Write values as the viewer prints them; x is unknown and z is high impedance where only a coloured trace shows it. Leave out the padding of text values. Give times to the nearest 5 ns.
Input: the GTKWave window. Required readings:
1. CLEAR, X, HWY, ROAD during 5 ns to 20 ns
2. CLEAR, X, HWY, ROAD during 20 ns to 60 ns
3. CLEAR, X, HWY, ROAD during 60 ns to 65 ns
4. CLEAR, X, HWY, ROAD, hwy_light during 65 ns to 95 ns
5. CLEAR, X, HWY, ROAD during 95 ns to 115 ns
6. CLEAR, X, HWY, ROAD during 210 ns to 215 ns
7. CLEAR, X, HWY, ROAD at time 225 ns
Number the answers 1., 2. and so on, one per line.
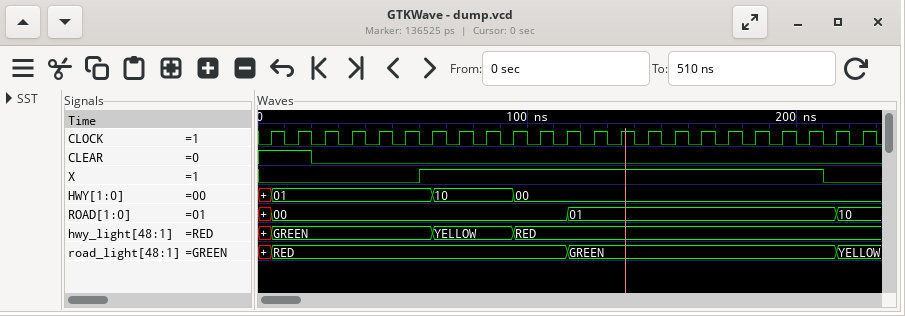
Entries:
1. CLEAR=1, X=0, HWY=01, ROAD=00
2. CLEAR=0, X=0, HWY=01, ROAD=00
3. CLEAR=0, X=1, HWY=01, ROAD=00
4. CLEAR=0, X=1, HWY=10, ROAD=00, hwy_light=YELLOW
5. CLEAR=0, X=1, HWY=00, ROAD=00
6. CLEAR=0, X=0, HWY=00, ROAD=01
7. CLEAR=0, X=0, HWY=00, ROAD=10
